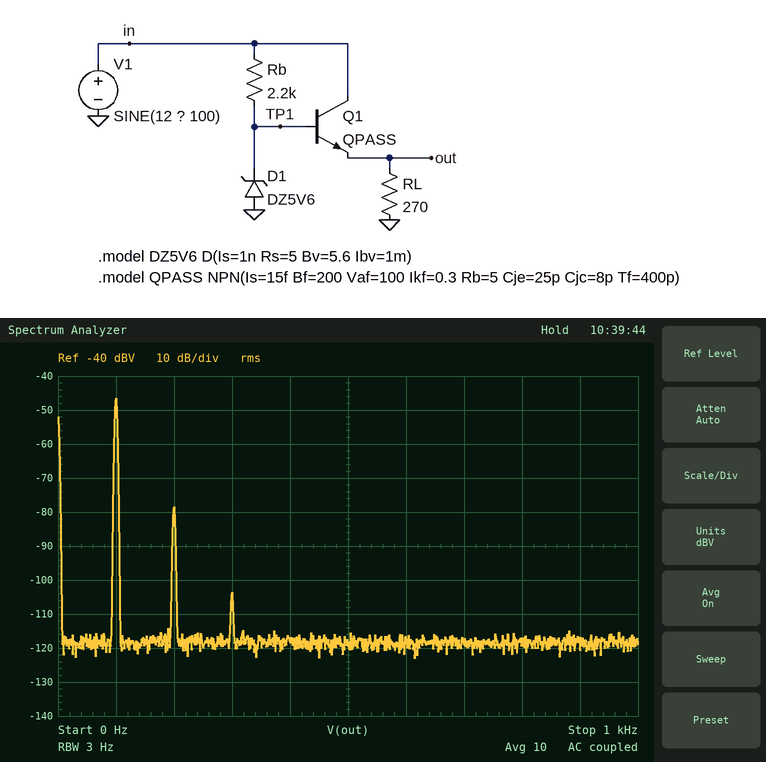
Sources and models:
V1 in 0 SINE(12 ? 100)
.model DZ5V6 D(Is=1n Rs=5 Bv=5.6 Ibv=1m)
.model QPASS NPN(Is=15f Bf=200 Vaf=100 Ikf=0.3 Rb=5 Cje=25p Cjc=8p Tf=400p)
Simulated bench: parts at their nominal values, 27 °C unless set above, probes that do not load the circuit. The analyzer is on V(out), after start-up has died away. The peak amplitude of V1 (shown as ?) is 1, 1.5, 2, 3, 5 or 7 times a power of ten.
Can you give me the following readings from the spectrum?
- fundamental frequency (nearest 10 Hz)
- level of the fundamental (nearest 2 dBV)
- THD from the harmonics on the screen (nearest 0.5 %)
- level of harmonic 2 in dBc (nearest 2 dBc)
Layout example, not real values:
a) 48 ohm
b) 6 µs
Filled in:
a) 100 Hz
b) -46 dBV
c) 2.5 %
d) -32 dBc
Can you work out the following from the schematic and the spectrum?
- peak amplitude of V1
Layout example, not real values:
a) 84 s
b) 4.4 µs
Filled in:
a) 1 V
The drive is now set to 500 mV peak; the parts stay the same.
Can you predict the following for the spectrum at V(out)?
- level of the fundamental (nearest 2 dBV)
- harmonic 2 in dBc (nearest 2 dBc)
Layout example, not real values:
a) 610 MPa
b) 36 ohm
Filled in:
a) -52 dBV
b) -38 dBc
